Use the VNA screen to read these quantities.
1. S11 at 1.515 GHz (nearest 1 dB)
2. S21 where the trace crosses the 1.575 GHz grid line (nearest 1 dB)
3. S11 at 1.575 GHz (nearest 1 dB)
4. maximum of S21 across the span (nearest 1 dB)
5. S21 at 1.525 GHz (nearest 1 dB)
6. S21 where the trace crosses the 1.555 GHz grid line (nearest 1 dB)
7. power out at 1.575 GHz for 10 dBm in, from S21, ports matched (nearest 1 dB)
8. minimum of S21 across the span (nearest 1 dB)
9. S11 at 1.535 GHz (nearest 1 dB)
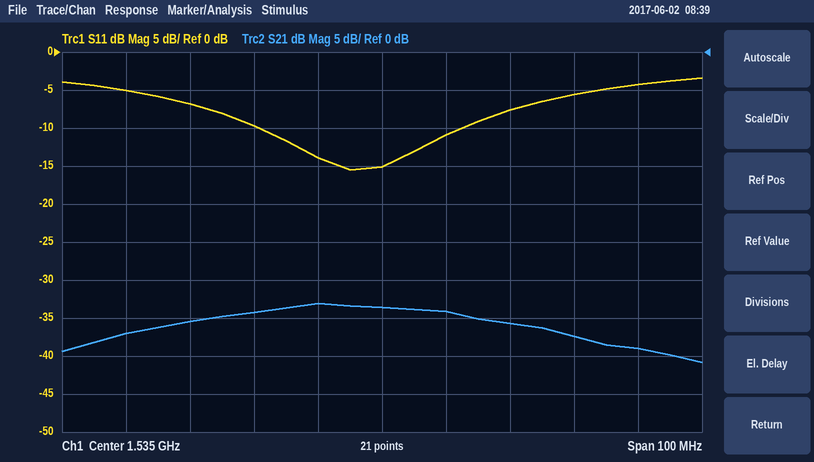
-10 dB
-39 dB
-4 dB
-33 dB
-33 dB
-36 dB
-29 dBm
-41 dB
-15 dB
